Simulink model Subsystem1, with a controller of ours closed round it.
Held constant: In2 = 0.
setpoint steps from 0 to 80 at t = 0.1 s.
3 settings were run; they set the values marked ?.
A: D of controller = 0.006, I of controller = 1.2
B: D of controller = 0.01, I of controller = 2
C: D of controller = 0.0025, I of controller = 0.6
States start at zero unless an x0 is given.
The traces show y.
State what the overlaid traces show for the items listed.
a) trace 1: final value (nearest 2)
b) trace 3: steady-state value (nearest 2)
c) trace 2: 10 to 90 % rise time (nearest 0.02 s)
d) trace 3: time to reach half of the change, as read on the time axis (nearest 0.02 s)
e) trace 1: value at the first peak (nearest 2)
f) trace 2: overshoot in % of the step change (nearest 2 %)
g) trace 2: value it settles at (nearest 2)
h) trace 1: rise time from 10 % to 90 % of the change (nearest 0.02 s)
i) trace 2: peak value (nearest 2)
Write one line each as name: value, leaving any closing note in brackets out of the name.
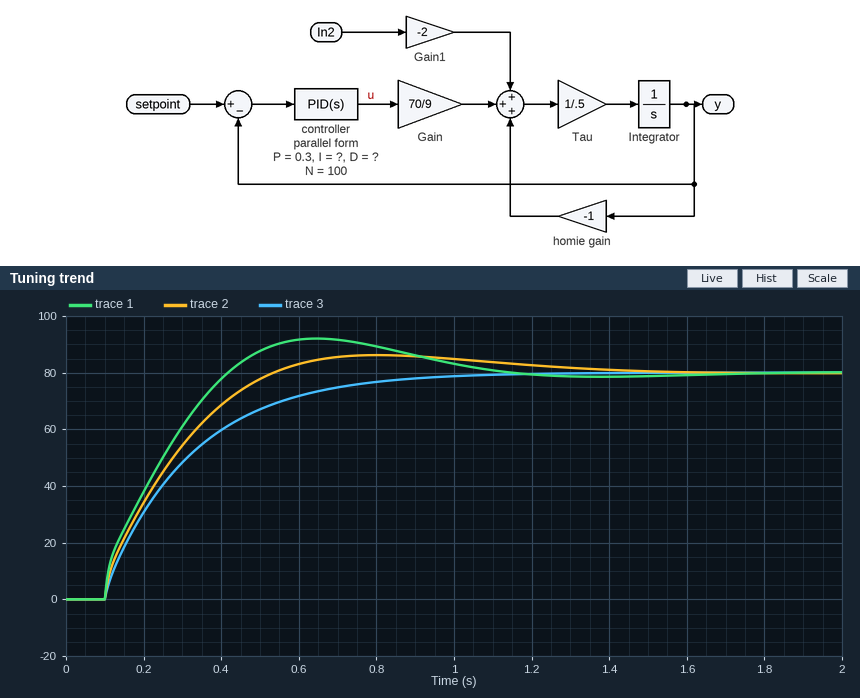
trace 1: final value: 80
trace 3: steady-state value: 80
trace 2: 10 to 90 % rise time: 0.32 s
trace 3: time to reach half of the change, as read on the time axis: 0.24 s
trace 1: value at the first peak: 92
trace 2: overshoot in % of the step change: 8 %
trace 2: value it settles at: 80
trace 1: rise time from 10 % to 90 % of the change: 0.26 s
trace 2: peak value: 86
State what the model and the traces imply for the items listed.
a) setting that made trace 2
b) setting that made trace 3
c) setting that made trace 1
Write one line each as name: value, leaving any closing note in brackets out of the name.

setting that made trace 2: A
setting that made trace 3: C
setting that made trace 1: B
